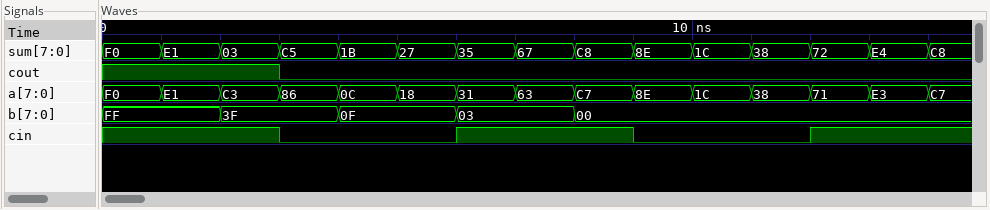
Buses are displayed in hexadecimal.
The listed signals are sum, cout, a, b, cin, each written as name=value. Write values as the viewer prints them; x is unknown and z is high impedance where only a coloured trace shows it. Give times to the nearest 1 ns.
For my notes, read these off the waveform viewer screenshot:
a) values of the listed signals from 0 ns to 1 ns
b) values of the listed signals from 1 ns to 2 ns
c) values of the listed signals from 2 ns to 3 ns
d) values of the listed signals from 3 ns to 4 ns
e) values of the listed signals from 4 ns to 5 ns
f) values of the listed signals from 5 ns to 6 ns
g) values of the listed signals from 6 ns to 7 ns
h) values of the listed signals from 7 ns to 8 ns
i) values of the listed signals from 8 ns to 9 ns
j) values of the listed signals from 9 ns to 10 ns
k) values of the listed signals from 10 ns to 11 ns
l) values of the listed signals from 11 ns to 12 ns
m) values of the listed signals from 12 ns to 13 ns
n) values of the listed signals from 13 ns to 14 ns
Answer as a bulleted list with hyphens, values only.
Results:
- sum=F0, cout=1, a=F0, b=FF, cin=1
- sum=E1, cout=1, a=E1, b=FF, cin=1
- sum=03, cout=1, a=C3, b=3F, cin=1
- sum=C5, cout=0, a=86, b=3F, cin=0
- sum=1B, cout=0, a=0C, b=0F, cin=0
- sum=27, cout=0, a=18, b=0F, cin=0
- sum=35, cout=0, a=31, b=03, cin=1
- sum=67, cout=0, a=63, b=03, cin=1
- sum=C8, cout=0, a=C7, b=00, cin=1
- sum=8E, cout=0, a=8E, b=00, cin=0
- sum=1C, cout=0, a=1C, b=00, cin=0
- sum=38, cout=0, a=38, b=00, cin=0
- sum=72, cout=0, a=71, b=00, cin=1
- sum=E4, cout=0, a=E3, b=00, cin=1
